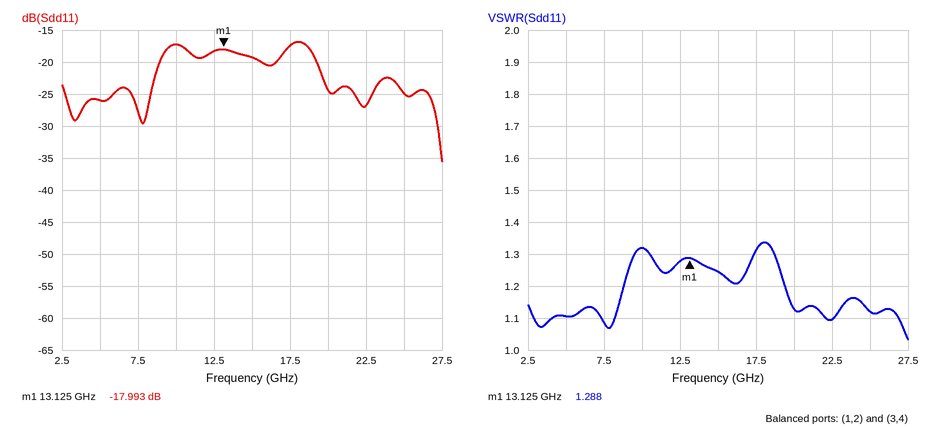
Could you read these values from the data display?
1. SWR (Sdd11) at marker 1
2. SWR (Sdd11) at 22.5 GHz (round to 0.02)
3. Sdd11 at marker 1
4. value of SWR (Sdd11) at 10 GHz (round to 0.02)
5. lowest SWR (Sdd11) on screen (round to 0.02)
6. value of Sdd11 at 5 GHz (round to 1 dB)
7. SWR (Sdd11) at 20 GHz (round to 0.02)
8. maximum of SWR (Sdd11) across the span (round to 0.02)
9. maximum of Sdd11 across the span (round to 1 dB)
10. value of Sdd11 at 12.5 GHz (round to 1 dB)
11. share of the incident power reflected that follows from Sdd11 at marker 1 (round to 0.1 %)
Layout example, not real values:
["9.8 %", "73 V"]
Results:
["1.288", "1.10", "-17.993 dB", "1.32", "1.04", "-26 dB", "1.12", "1.34", "-17 dB", "-18 dB", "1.6 %"]
